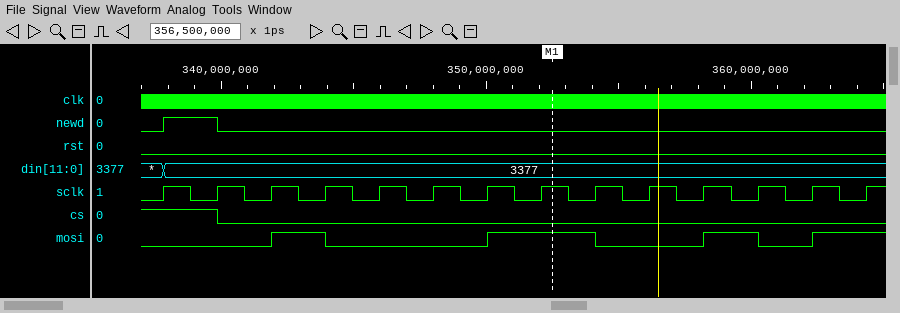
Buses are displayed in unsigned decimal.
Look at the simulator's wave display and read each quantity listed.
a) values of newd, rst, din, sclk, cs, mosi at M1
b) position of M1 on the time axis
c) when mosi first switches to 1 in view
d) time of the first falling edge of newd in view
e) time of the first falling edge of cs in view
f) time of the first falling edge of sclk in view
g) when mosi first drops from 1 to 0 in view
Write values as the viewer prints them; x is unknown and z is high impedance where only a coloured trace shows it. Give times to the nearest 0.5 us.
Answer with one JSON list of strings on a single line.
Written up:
["newd=0, rst=0, din=3377, sclk=1, cs=0, mosi=1", "352.5 us", "342 us", "340 us", "340 us", "339 us", "344 us"]
